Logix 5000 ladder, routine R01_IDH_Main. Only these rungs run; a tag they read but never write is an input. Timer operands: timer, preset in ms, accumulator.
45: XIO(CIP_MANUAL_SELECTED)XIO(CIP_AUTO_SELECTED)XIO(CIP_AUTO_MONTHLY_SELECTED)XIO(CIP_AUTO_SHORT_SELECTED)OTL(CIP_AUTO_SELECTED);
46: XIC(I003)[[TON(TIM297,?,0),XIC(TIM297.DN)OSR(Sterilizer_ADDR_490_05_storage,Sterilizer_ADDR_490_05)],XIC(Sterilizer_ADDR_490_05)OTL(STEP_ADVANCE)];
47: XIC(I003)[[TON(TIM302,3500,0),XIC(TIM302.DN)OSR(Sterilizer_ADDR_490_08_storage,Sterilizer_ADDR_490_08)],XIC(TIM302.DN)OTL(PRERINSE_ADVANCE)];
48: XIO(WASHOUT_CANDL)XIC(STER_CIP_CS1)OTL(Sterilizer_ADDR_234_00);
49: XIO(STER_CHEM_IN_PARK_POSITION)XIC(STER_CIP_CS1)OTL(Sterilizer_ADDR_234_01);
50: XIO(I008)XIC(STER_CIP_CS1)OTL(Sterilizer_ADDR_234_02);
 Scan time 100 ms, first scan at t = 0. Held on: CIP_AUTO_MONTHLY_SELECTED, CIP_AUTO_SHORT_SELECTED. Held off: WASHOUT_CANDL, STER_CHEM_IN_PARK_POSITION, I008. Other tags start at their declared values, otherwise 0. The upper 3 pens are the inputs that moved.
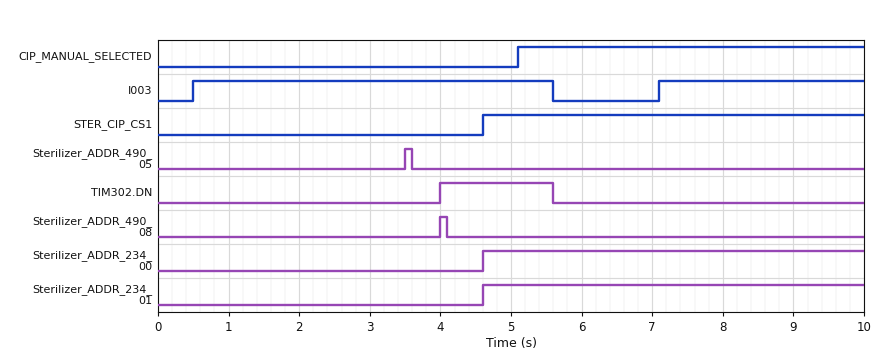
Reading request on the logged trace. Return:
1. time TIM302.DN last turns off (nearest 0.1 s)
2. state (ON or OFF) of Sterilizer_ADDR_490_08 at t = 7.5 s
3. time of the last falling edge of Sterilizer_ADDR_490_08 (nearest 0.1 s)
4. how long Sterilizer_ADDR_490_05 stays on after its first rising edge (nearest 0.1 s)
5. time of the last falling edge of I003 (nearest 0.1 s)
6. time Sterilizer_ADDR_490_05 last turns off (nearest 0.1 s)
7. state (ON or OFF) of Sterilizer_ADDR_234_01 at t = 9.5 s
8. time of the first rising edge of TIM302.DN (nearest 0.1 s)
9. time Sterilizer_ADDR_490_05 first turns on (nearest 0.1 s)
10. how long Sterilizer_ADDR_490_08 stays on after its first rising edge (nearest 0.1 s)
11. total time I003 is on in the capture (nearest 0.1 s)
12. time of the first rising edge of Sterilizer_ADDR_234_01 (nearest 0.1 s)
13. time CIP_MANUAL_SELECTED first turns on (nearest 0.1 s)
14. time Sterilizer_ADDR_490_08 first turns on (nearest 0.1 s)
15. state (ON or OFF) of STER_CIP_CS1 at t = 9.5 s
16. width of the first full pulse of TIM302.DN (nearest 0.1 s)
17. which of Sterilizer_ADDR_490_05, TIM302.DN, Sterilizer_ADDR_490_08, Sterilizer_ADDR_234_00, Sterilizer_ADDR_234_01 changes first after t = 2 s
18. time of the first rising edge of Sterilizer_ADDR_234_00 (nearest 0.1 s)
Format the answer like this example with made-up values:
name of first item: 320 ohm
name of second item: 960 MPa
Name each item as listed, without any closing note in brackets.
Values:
time TIM302.DN last turns off: 5.6 s
state (ON or OFF) of Sterilizer_ADDR_490_08 at t = 7.5 s: OFF
time of the last falling edge of Sterilizer_ADDR_490_08: 4.1 s
how long Sterilizer_ADDR_490_05 stays on after its first rising edge: 0.1 s
time of the last falling edge of I003: 5.6 s
time Sterilizer_ADDR_490_05 last turns off: 3.6 s
state (ON or OFF) of Sterilizer_ADDR_234_01 at t = 9.5 s: ON
time of the first rising edge of TIM302.DN: 4.0 s
time Sterilizer_ADDR_490_05 first turns on: 3.5 s
how long Sterilizer_ADDR_490_08 stays on after its first rising edge: 0.1 s
total time I003 is on in the capture: 8.0 s
time of the first rising edge of Sterilizer_ADDR_234_01: 4.6 s
time CIP_MANUAL_SELECTED first turns on: 5.1 s
time Sterilizer_ADDR_490_08 first turns on: 4.0 s
state (ON or OFF) of STER_CIP_CS1 at t = 9.5 s: ON
width of the first full pulse of TIM302.DN: 1.6 s
which of Sterilizer_ADDR_490_05, TIM302.DN, Sterilizer_ADDR_490_08, Sterilizer_ADDR_234_00, Sterilizer_ADDR_234_01 changes first after t = 2 s: Sterilizer_ADDR_490_05
time of the first rising edge of Sterilizer_ADDR_234_00: 4.6 s
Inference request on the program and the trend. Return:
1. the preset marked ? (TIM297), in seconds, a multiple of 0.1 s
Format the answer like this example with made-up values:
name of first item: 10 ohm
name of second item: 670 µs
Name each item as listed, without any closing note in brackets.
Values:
the preset marked ? (TIM297), in seconds, a multiple of 0.1 s: 3.0 s
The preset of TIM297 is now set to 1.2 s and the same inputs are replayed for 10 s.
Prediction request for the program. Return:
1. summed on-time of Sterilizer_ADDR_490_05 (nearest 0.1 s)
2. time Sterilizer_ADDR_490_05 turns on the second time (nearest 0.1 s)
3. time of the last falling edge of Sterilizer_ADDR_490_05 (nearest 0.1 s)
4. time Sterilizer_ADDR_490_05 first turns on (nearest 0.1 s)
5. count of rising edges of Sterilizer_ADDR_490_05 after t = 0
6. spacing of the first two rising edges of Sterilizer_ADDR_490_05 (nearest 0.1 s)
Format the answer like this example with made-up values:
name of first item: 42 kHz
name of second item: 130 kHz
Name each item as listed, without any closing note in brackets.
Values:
summed on-time of Sterilizer_ADDR_490_05: 0.2 s
time Sterilizer_ADDR_490_05 turns on the second time: 8.3 s
time of the last falling edge of Sterilizer_ADDR_490_05: 8.4 s
time Sterilizer_ADDR_490_05 first turns on: 1.7 s
count of rising edges of Sterilizer_ADDR_490_05 after t = 0: 2
spacing of the first two rising edges of Sterilizer_ADDR_490_05: 6.6 s
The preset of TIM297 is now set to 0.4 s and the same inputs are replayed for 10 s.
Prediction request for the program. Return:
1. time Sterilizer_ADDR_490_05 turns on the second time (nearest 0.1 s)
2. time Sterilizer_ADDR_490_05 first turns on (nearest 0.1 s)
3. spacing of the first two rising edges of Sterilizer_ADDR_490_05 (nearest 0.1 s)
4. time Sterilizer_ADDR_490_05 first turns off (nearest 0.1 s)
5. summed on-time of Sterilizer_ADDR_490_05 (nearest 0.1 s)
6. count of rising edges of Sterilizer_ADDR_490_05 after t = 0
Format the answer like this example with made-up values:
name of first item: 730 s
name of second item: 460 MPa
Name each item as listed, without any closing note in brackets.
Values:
time Sterilizer_ADDR_490_05 turns on the second time: 7.5 s
time Sterilizer_ADDR_490_05 first turns on: 0.9 s
spacing of the first two rising edges of Sterilizer_ADDR_490_05: 6.6 s
time Sterilizer_ADDR_490_05 first turns off: 1.0 s
summed on-time of Sterilizer_ADDR_490_05: 0.2 s
count of rising edges of Sterilizer_ADDR_490_05 after t = 0: 2
